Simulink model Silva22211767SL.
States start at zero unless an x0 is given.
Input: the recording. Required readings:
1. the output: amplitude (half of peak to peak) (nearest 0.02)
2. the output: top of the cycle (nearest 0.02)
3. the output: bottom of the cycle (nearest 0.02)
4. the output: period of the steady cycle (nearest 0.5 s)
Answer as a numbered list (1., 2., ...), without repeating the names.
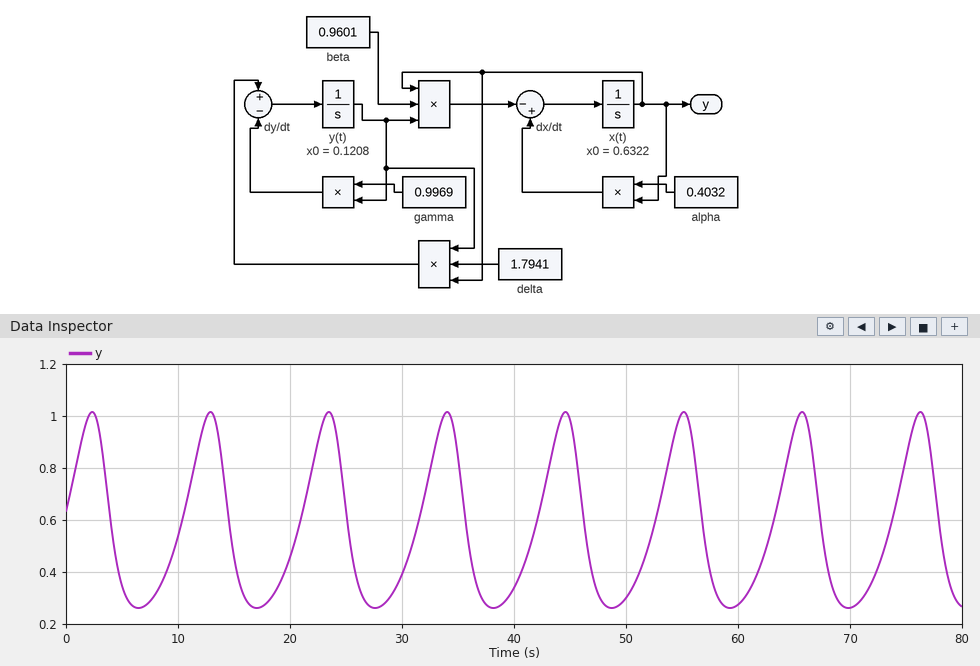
1. 0.38
2. 1.02
3. 0.26
4. 10.5 s
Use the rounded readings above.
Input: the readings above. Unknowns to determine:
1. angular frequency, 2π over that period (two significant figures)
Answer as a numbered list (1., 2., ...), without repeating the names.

1. 0.60 rad/s
